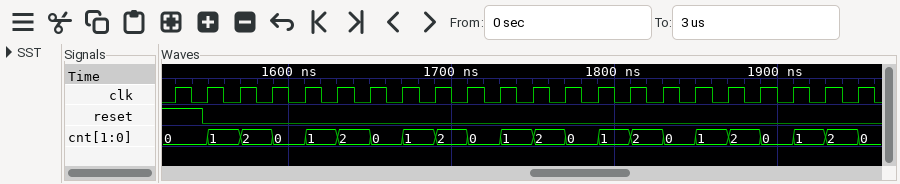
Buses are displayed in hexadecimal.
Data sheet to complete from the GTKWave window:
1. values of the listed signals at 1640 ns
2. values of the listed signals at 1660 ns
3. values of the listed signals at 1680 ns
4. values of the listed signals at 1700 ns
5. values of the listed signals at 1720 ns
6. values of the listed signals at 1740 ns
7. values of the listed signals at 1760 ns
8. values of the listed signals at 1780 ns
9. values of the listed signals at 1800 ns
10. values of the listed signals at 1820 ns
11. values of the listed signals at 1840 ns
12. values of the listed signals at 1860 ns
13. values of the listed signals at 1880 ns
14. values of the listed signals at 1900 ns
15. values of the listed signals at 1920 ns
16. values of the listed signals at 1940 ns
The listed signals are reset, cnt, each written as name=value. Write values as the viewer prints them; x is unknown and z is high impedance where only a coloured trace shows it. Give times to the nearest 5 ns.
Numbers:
reset=0, cnt=2
reset=0, cnt=0
reset=0, cnt=1
reset=0, cnt=2
reset=0, cnt=0
reset=0, cnt=1
reset=0, cnt=2
reset=0, cnt=0
reset=0, cnt=1
reset=0, cnt=2
reset=0, cnt=0
reset=0, cnt=1
reset=0, cnt=2
reset=0, cnt=0
reset=0, cnt=1
reset=0, cnt=2
